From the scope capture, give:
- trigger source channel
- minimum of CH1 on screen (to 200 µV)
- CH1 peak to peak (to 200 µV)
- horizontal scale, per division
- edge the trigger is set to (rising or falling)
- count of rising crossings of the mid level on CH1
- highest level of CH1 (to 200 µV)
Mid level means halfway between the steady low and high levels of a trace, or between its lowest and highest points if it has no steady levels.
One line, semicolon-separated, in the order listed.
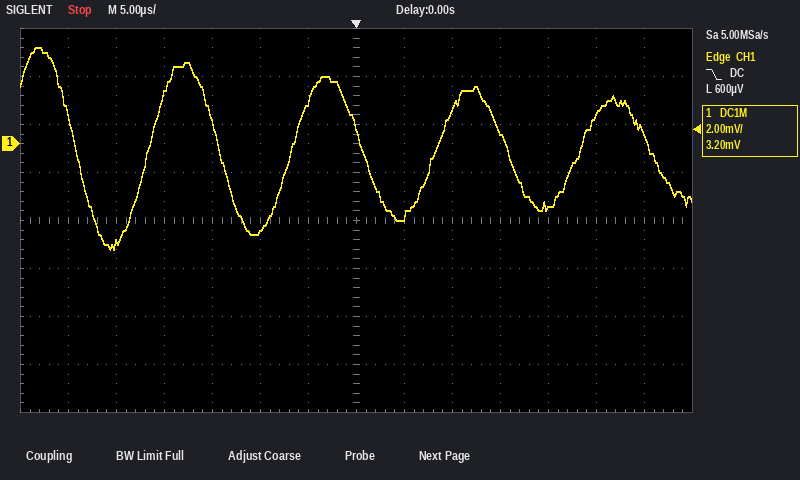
CH1; -4.4 mV; 8.4 mV; 5 µs; falling; 4; 4.0 mV
